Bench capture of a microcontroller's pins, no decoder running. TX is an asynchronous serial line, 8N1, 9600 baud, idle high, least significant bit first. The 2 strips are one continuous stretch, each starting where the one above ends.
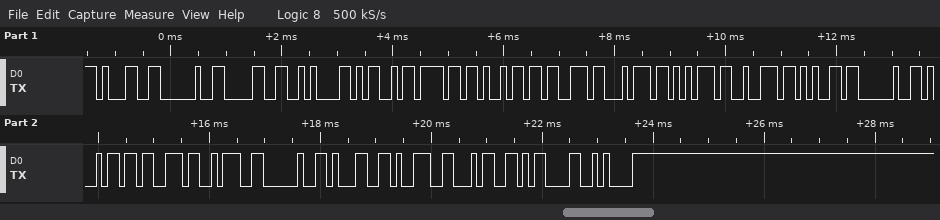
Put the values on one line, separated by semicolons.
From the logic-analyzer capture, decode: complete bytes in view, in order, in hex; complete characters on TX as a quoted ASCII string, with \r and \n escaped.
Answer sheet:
0x31 0x20 0x30 0x0A 0x4D 0x6F 0x69 0x73 0x74 0x75 0x72 0x65 0x20 0x69 0x73 0x3A 0x20 0x31 0x39 0x34 0x0D 0x0A; "1 0\nMoisture is: 194\r\n"
